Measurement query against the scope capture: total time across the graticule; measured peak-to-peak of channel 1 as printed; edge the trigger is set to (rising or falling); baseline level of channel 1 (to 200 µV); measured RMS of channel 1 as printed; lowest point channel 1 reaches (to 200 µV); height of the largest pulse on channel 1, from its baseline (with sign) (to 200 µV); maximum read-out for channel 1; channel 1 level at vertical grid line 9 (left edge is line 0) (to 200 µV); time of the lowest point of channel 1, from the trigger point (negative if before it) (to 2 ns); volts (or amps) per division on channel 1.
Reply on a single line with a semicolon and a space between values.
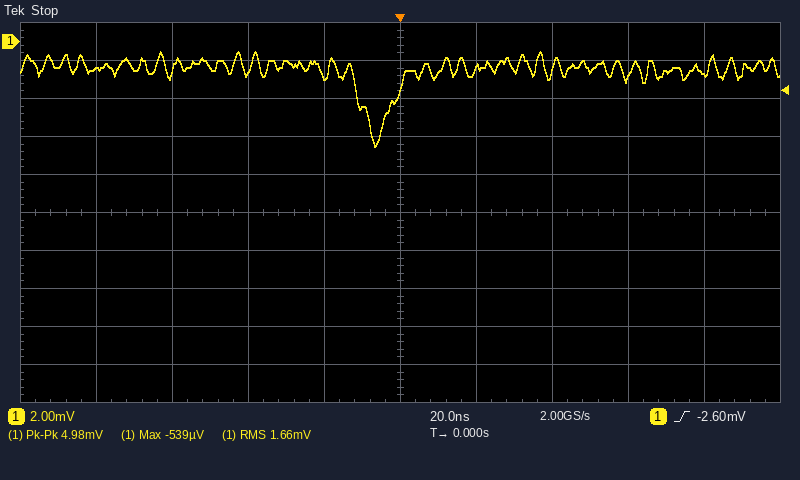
200 ns; 4.98 mV; rising; -1.4 mV; 1.66 mV; -5.6 mV; -4.2 mV; -539 µV; -1.6 mV; -6 ns; 2 mV
